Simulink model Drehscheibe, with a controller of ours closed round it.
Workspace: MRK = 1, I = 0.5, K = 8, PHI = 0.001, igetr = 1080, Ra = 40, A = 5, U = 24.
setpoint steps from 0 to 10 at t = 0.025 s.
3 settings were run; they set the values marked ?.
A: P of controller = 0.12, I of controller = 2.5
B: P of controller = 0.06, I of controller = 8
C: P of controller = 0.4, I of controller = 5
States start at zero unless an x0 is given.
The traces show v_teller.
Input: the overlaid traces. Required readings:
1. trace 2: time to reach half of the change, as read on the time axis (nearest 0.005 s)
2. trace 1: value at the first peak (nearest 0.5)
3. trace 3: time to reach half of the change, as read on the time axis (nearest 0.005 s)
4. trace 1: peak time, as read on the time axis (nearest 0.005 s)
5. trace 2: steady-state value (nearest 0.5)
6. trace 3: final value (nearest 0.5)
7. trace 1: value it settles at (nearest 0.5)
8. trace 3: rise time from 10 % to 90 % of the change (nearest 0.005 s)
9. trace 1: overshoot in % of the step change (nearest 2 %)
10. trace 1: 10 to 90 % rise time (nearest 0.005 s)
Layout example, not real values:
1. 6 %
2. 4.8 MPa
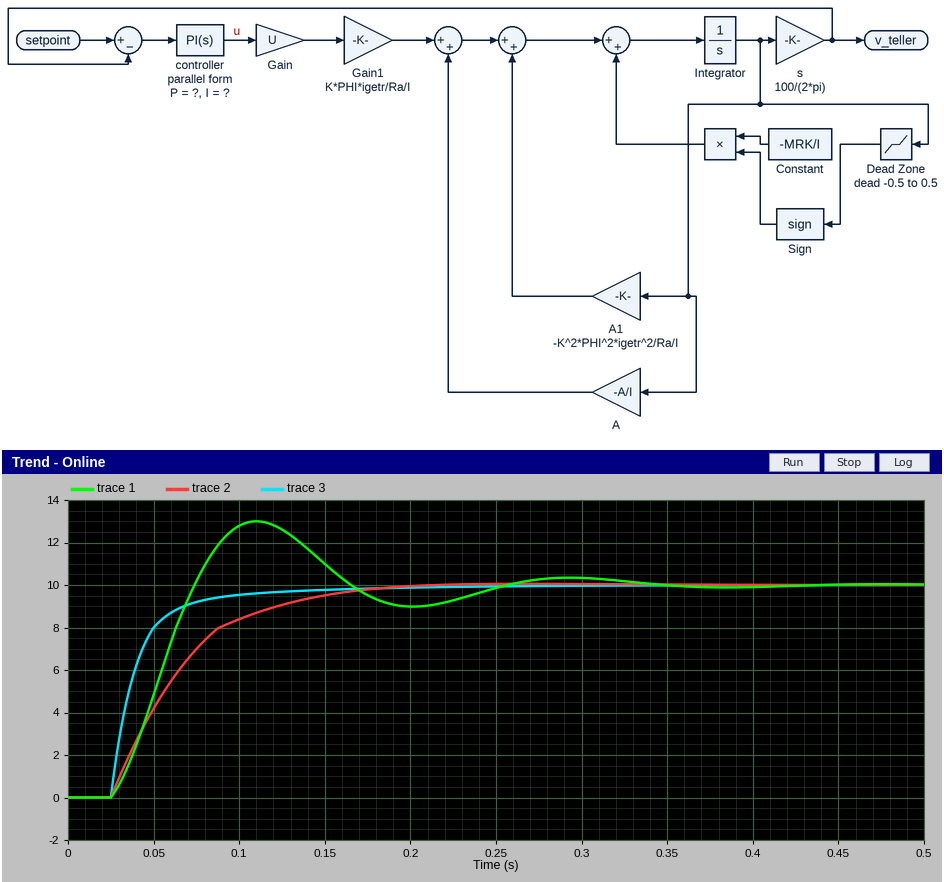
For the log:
1. 0.055 s
2. 13.0
3. 0.035 s
4. 0.110 s
5. 10.0
6. 10.0
7. 10.0
8. 0.040 s
9. 30 %
10. 0.035 s
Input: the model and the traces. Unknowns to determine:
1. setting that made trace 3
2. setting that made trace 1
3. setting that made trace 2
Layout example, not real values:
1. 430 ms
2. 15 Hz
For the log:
1. C
2. B
3. A
